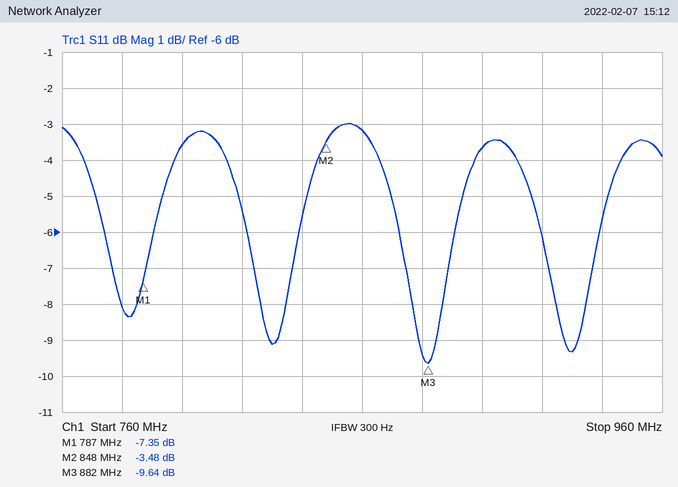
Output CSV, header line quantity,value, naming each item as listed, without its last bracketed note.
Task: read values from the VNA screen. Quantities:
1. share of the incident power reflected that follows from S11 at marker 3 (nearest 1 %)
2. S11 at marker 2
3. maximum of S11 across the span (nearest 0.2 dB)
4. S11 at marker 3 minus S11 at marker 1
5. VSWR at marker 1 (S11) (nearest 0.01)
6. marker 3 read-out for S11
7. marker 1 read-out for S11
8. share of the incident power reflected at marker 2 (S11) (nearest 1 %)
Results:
quantity,value
share of the incident power reflected that follows from S11 at marker 3,11 %
S11 at marker 2,-3.48 dB
maximum of S11 across the span,-3.0 dB
S11 at marker 3 minus S11 at marker 1,-2.29 dB
VSWR at marker 1 (S11),2.50
marker 3 read-out for S11,-9.64 dB
marker 1 read-out for S11,-7.35 dB
share of the incident power reflected at marker 2 (S11),45 %
